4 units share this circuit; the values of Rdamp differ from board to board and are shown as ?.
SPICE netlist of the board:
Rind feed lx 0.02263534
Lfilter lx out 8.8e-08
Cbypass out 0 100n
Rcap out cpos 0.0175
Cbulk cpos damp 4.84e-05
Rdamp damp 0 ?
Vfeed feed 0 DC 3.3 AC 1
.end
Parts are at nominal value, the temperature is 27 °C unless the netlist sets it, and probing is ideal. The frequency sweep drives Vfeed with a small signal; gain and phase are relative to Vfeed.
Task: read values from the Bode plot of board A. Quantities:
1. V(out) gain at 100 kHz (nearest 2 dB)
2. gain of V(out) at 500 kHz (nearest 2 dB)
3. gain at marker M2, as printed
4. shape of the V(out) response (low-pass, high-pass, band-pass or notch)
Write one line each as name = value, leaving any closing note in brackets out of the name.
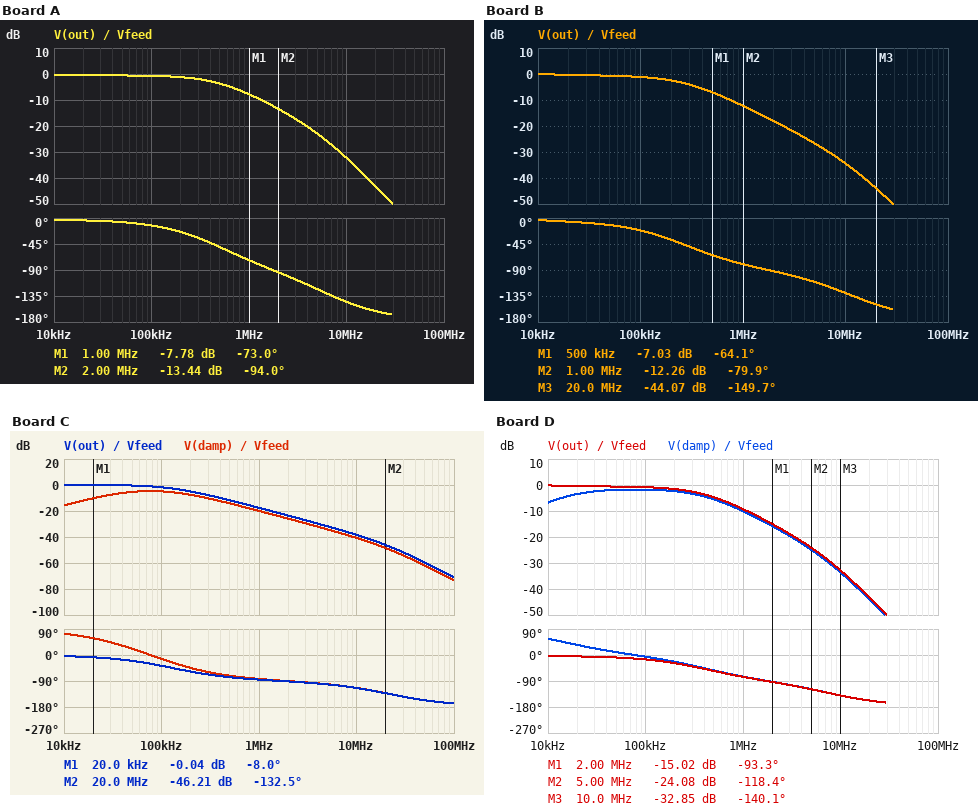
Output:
V(out) gain at 100 kHz = 0 dB
gain of V(out) at 500 kHz = -4 dB
gain at marker M2, as printed = -13.44 dB
shape of the V(out) response = low-pass
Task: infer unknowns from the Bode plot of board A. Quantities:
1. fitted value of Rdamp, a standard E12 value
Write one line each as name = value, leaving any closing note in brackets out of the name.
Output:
fitted value of Rdamp, a standard E12 value = 0.22 Ω
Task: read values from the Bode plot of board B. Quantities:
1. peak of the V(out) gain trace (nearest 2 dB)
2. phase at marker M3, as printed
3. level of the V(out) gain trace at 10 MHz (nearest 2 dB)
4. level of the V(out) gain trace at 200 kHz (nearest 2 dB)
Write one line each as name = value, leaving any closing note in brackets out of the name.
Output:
peak of the V(out) gain trace = 0 dB
phase at marker M3, as printed = -149.7 deg
level of the V(out) gain trace at 10 MHz = -34 dB
level of the V(out) gain trace at 200 kHz = -2 dB
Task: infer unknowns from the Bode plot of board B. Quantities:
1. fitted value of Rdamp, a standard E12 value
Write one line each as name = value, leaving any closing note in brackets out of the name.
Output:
fitted value of Rdamp, a standard E12 value = 0.12 Ω
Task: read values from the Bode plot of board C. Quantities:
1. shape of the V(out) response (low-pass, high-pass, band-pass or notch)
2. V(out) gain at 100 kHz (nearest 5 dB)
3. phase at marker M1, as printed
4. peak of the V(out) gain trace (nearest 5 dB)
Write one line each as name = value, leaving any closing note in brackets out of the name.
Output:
shape of the V(out) response = low-pass
V(out) gain at 100 kHz = 0 dB
phase at marker M1, as printed = -8.0 deg
peak of the V(out) gain trace = 0 dB
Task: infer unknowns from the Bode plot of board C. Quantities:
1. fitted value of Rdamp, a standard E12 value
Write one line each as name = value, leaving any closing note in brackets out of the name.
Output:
fitted value of Rdamp, a standard E12 value = 0.056 Ω
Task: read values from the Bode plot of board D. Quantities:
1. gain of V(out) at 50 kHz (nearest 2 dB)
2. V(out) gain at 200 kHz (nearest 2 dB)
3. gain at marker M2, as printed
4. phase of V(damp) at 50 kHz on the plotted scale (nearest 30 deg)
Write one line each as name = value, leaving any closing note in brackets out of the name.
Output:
gain of V(out) at 50 kHz = 0 dB
V(out) gain at 200 kHz = -2 dB
gain at marker M2, as printed = -24.08 dB
phase of V(damp) at 50 kHz on the plotted scale = 0 deg
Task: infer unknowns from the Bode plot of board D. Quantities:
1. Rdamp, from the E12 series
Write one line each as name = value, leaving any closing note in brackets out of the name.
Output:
Rdamp, from the E12 series = 0.18 Ω
